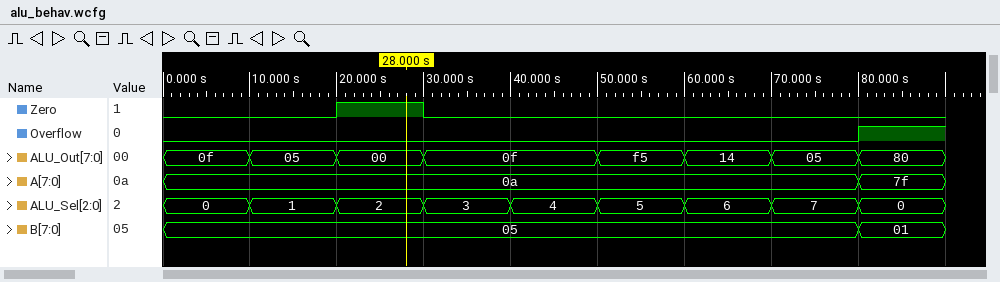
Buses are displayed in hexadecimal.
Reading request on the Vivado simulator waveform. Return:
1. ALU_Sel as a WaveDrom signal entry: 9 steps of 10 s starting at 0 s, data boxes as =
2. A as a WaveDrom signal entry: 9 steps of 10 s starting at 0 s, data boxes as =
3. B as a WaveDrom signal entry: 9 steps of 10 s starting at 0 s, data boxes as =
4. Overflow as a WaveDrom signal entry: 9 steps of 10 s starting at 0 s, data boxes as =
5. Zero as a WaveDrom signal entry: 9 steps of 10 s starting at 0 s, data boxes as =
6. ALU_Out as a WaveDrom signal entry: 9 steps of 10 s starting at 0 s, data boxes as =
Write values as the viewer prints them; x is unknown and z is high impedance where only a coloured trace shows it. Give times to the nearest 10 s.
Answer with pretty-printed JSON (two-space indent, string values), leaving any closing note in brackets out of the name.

{
  "ALU_Sel as a WaveDrom signal entry: 9 steps of 10 s starting at 0 s, data boxes as =": "{name: 'ALU_Sel', wave: '=========', data: '0 1 2 3 4 5 6 7 0'}",
  "A as a WaveDrom signal entry: 9 steps of 10 s starting at 0 s, data boxes as =": "{name: 'A', wave: '=.......=', data: '0a 7f'}",
  "B as a WaveDrom signal entry: 9 steps of 10 s starting at 0 s, data boxes as =": "{name: 'B', wave: '=.......=', data: '05 01'}",
  "Overflow as a WaveDrom signal entry: 9 steps of 10 s starting at 0 s, data boxes as =": "{name: 'Overflow', wave: '0.......1'}",
  "Zero as a WaveDrom signal entry: 9 steps of 10 s starting at 0 s, data boxes as =": "{name: 'Zero', wave: '0.10.....'}",
  "ALU_Out as a WaveDrom signal entry: 9 steps of 10 s starting at 0 s, data boxes as =": "{name: 'ALU_Out', wave: '====.====', data: '0f 05 00 0f f5 14 05 80'}"
}
